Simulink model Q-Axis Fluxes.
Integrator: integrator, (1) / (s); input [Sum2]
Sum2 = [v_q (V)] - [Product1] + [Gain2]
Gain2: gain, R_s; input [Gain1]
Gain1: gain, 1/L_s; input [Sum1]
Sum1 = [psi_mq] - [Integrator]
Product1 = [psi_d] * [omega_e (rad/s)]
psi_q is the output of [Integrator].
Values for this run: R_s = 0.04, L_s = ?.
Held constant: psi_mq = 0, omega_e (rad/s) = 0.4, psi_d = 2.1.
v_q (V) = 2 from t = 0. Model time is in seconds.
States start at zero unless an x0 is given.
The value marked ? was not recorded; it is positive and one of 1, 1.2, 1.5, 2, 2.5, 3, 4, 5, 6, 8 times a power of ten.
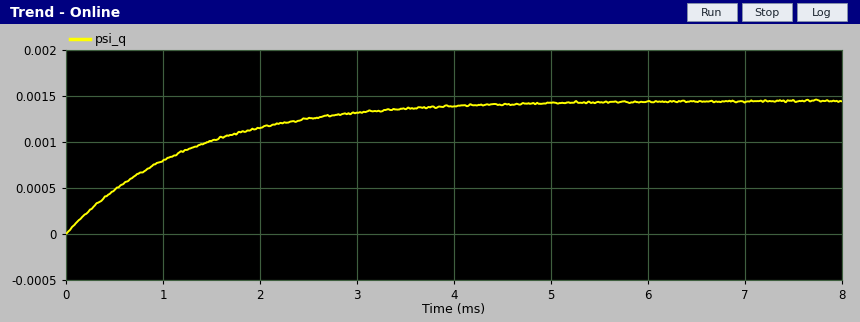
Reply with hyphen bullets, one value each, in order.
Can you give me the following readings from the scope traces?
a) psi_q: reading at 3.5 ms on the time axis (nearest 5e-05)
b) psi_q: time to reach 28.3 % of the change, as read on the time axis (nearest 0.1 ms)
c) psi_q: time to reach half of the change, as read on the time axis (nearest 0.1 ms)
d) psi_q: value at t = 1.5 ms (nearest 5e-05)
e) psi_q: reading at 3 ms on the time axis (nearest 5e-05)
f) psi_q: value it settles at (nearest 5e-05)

- 0.00135
- 0.4 ms
- 0.9 ms
- 0.00100
- 0.00130
- 0.00145
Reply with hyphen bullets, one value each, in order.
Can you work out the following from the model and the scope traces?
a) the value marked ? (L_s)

- 5e-05
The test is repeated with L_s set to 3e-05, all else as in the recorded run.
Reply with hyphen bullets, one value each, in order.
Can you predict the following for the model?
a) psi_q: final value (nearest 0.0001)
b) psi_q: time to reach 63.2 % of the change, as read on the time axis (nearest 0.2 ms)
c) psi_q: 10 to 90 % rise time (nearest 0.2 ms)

- 0.0009
- 0.8 ms
- 1.6 ms
